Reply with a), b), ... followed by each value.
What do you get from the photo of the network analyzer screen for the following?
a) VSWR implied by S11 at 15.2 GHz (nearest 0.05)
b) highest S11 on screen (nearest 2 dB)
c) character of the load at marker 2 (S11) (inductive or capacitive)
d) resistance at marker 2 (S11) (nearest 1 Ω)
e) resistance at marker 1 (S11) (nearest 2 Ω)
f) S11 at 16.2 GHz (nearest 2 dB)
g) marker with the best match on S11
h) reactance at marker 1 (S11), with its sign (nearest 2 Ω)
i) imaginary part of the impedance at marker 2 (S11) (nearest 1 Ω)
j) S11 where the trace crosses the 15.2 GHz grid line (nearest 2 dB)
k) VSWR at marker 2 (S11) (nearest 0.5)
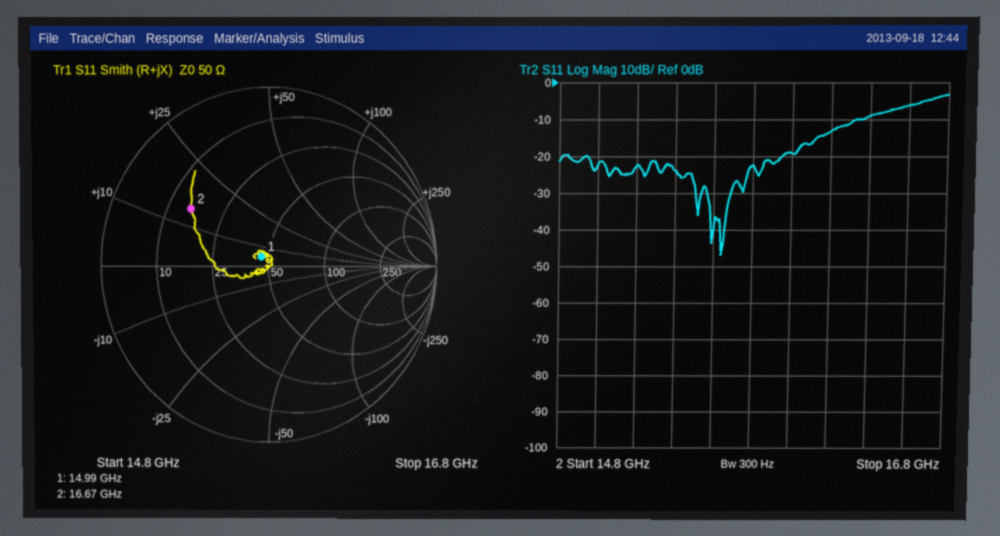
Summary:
a) 1.15
b) -4 dB
c) inductive
d) 15 Ω
e) 46 Ω
f) -14 dB
g) marker 1
h) +4 Ω
i) +14 Ω
j) -22 dB
k) 3.5
